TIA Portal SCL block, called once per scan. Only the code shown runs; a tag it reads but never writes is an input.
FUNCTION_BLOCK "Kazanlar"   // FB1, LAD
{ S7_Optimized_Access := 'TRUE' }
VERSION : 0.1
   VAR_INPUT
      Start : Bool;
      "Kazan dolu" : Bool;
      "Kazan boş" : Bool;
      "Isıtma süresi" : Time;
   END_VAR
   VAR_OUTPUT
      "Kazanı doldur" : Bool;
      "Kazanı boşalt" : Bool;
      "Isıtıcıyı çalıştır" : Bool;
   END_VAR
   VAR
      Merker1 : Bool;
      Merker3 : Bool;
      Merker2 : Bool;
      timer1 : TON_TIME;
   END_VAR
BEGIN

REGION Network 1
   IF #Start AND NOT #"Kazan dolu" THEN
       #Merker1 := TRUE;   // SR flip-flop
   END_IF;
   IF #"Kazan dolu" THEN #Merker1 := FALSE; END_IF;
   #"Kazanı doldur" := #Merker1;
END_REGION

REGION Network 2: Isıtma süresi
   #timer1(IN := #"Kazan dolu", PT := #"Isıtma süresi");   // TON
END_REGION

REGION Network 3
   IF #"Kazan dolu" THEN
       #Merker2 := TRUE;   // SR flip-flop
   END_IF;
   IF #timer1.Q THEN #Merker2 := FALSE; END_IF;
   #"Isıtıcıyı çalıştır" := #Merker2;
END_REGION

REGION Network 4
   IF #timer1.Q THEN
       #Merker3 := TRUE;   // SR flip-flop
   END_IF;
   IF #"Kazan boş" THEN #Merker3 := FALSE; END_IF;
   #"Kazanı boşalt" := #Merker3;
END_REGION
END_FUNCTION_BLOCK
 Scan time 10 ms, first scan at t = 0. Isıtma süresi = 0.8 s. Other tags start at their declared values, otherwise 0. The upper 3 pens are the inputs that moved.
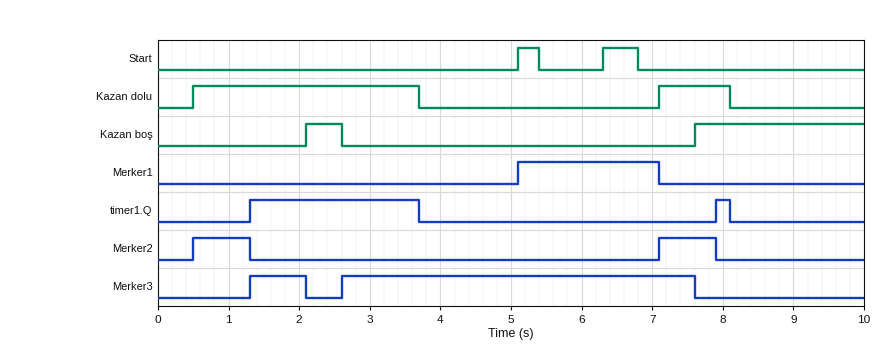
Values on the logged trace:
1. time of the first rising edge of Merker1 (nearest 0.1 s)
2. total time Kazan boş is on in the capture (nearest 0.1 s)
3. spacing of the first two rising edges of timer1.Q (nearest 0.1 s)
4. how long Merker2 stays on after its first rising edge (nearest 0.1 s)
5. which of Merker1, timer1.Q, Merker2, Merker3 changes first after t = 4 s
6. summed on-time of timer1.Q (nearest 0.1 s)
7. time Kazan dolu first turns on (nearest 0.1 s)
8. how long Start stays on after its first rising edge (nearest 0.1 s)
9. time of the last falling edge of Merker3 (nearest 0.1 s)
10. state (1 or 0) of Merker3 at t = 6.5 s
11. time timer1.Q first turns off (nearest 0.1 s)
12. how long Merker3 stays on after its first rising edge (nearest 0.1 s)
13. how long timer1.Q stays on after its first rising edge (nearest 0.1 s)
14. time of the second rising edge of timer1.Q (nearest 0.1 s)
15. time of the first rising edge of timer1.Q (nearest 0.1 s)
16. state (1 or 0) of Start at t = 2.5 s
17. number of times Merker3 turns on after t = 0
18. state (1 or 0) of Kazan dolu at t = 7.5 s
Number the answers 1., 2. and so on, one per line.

1. 5.1 s
2. 2.9 s
3. 6.6 s
4. 0.8 s
5. Merker1
6. 2.6 s
7. 0.5 s
8. 0.3 s
9. 7.6 s
10. 1
11. 3.7 s
12. 0.8 s
13. 2.4 s
14. 7.9 s
15. 1.3 s
16. 0
17. 2
18. 1
